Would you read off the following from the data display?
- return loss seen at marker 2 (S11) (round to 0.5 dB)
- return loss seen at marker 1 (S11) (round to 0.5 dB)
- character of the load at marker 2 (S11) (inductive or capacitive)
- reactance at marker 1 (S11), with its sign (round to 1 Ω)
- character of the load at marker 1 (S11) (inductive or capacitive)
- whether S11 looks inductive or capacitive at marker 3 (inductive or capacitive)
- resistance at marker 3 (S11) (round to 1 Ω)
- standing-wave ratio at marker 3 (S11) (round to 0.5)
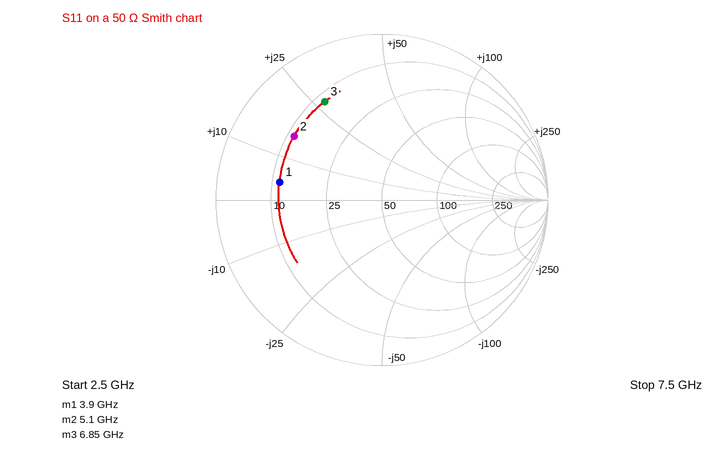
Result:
3.5 dB
4.0 dB
inductive
+4 Ω
inductive
inductive
12 Ω
5.5
